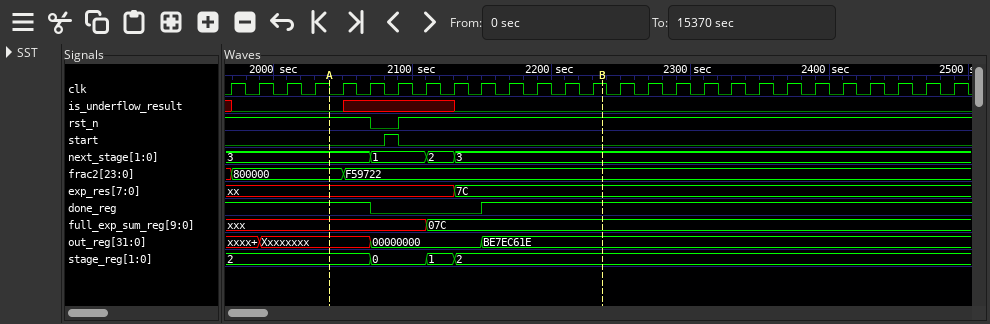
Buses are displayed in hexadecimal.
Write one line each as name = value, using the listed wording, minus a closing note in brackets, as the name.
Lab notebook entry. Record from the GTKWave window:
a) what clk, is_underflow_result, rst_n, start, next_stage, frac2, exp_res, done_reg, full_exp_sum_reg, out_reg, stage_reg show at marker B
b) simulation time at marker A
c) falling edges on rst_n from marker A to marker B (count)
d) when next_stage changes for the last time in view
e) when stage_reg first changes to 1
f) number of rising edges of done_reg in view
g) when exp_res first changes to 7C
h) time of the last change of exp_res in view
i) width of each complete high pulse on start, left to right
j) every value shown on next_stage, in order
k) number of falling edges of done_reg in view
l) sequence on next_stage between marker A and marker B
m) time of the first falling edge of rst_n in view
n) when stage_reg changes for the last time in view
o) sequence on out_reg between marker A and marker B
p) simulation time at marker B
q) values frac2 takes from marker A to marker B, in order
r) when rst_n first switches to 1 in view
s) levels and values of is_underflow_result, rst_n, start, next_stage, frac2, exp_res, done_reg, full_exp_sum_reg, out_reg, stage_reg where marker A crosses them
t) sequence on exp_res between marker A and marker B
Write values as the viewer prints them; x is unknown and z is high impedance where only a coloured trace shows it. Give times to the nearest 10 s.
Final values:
what clk, is_underflow_result, rst_n, start, next_stage, frac2, exp_res, done_reg, full_exp_sum_reg, out_reg, stage_reg show at marker B = clk=1, is_underflow_result=0, rst_n=1, start=0, next_stage=3, frac2=F59722, exp_res=7C, done_reg=1, full_exp_sum_reg=07C, out_reg=BE7EC61E, stage_reg=2
simulation time at marker A = 2040 s
falling edges on rst_n from marker A to marker B = 1
when next_stage changes for the last time in view = 2130 s
when stage_reg first changes to 1 = 2110 s
number of rising edges of done_reg in view = 1
when exp_res first changes to 7C = 2130 s
time of the last change of exp_res in view = 2130 s
width of each complete high pulse on start, left to right = 10 s
every value shown on next_stage, in order = 3, 1, 2, 3
number of falling edges of done_reg in view = 1
sequence on next_stage between marker A and marker B = 3, 1, 2, 3
time of the first falling edge of rst_n in view = 2070 s
when stage_reg changes for the last time in view = 2130 s
sequence on out_reg between marker A and marker B = Xxxxxxxx, 00000000, BE7EC61E
simulation time at marker B = 2240 s
values frac2 takes from marker A to marker B, in order = 800000, F59722
when rst_n first switches to 1 in view = 2090 s
levels and values of is_underflow_result, rst_n, start, next_stage, frac2, exp_res, done_reg, full_exp_sum_reg, out_reg, stage_reg where marker A crosses them = is_underflow_result=0, rst_n=1, start=0, next_stage=3, frac2=800000, exp_res=xx, done_reg=1, full_exp_sum_reg=xxx, out_reg=Xxxxxxxx, stage_reg=2
sequence on exp_res between marker A and marker B = xx, 7C
